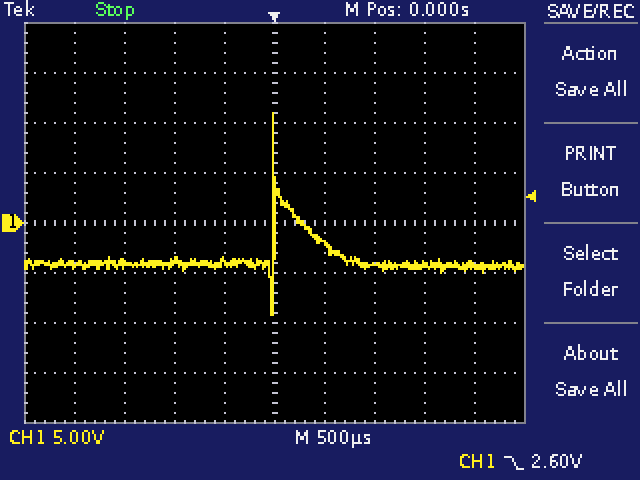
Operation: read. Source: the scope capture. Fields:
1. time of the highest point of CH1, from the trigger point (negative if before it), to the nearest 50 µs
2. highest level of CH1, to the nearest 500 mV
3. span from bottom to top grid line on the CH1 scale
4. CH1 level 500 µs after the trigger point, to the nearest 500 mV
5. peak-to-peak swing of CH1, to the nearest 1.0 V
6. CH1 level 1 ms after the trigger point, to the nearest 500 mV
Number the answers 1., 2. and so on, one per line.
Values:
1. 0 µs
2. 11.0 V
3. 40 V
4. -2.0 V
5. 20.0 V
6. -4.0 V
